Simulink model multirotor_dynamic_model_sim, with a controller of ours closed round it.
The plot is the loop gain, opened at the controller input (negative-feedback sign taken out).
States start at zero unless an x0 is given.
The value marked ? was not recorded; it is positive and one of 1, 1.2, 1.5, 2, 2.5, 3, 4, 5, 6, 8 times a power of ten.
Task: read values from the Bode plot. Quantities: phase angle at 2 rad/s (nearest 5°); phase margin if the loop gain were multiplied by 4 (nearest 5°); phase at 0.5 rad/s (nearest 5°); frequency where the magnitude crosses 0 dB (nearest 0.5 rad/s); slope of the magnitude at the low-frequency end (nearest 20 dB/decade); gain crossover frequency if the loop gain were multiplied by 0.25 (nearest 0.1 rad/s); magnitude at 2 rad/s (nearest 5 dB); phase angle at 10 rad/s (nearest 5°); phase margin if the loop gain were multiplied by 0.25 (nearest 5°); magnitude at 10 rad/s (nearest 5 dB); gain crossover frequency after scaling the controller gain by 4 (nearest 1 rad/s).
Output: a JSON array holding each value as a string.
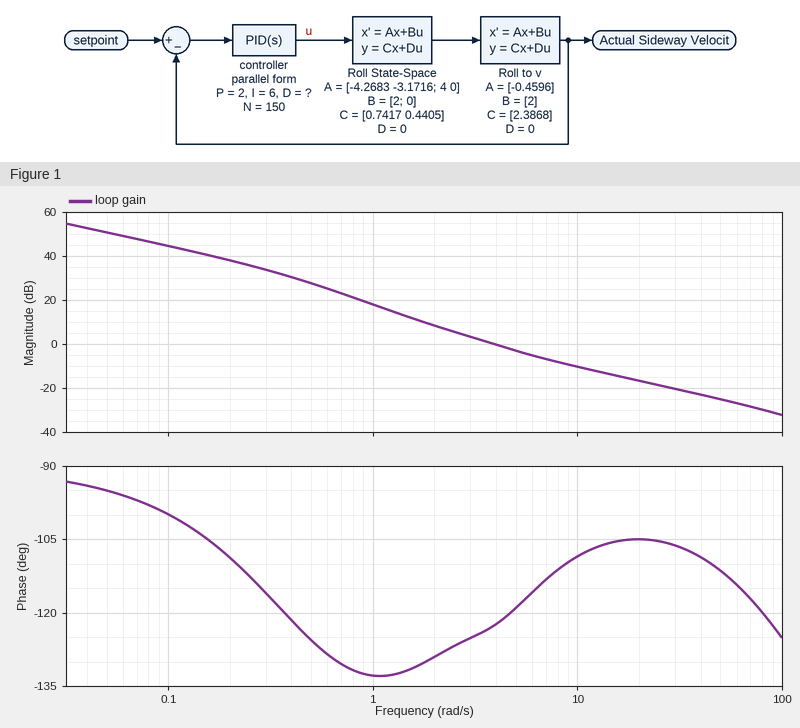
["-130°", "75°", "-125°", "4.0 rad/s", "-20 dB/decade", "1.5 rad/s", "10 dB", "-110°", "50°", "-10 dB", "12 rad/s"]
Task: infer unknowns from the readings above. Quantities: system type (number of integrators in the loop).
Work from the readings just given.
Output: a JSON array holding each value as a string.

["1"]
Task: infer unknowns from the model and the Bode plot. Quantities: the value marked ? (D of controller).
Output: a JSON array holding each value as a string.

["0.4"]
